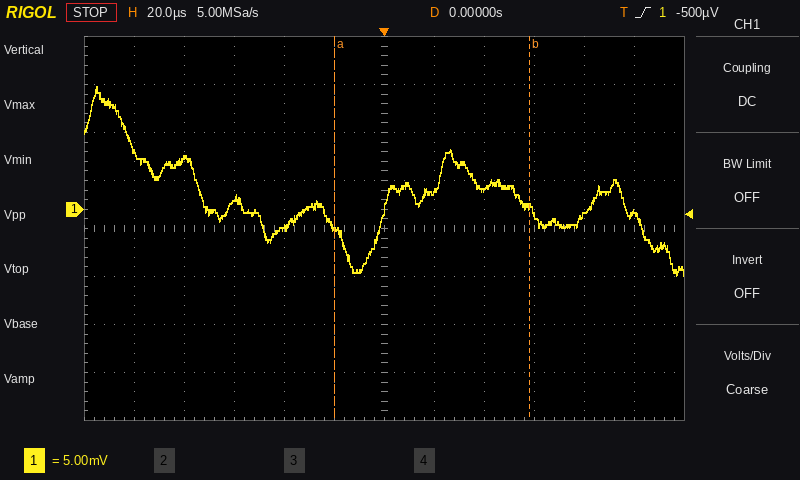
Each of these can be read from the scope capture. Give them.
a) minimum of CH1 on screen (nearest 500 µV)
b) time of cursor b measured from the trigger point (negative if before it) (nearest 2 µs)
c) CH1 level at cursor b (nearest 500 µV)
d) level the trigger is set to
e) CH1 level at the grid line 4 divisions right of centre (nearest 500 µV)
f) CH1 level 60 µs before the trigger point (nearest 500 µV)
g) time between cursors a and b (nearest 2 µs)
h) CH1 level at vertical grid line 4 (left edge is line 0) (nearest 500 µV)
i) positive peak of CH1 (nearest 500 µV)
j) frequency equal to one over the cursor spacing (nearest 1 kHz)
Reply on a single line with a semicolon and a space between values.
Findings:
-7.0 mV; +58 µs; 0.0 mV; -500 µV; -500 µV; 1.0 mV; 78 µs; -2.0 mV; 13.0 mV; 13 kHz
